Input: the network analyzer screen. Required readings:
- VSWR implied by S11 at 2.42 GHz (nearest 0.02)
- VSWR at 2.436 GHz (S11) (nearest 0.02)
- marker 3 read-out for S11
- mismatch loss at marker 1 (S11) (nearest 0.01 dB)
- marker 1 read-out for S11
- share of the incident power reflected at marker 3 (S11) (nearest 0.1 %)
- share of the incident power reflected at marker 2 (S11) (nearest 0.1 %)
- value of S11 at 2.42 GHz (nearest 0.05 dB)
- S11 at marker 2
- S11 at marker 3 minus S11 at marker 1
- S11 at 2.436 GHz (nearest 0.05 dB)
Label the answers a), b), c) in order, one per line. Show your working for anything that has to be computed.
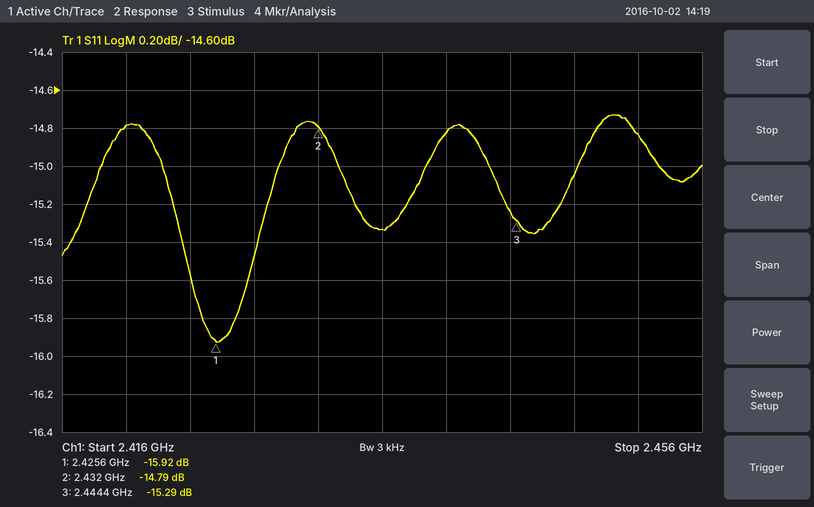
a) |Γ| = 10^(-14.8/20) = 0.1820; VSWR = (1 + 0.1820)/(1 − 0.1820) ≈ 1.44
b) |Γ| = 10^(-15.35/20) = 0.1708; VSWR = (1 + 0.1708)/(1 − 0.1708) ≈ 1.41, so 1.42 to the nearest 0.02
c) -15.29 dB
d) −10 log10(1 − 10^(-15.92/10)) ≈ 0.11 dB
e) -15.92 dB
f) 10^(-15.29/10) ≈ 3.0 %
g) 10^(-14.79/10) ≈ 3.3 %
h) -14.80 dB
i) -14.79 dB
j) -15.29 − (-15.92) = 0.63 dB
k) -15.35 dB
